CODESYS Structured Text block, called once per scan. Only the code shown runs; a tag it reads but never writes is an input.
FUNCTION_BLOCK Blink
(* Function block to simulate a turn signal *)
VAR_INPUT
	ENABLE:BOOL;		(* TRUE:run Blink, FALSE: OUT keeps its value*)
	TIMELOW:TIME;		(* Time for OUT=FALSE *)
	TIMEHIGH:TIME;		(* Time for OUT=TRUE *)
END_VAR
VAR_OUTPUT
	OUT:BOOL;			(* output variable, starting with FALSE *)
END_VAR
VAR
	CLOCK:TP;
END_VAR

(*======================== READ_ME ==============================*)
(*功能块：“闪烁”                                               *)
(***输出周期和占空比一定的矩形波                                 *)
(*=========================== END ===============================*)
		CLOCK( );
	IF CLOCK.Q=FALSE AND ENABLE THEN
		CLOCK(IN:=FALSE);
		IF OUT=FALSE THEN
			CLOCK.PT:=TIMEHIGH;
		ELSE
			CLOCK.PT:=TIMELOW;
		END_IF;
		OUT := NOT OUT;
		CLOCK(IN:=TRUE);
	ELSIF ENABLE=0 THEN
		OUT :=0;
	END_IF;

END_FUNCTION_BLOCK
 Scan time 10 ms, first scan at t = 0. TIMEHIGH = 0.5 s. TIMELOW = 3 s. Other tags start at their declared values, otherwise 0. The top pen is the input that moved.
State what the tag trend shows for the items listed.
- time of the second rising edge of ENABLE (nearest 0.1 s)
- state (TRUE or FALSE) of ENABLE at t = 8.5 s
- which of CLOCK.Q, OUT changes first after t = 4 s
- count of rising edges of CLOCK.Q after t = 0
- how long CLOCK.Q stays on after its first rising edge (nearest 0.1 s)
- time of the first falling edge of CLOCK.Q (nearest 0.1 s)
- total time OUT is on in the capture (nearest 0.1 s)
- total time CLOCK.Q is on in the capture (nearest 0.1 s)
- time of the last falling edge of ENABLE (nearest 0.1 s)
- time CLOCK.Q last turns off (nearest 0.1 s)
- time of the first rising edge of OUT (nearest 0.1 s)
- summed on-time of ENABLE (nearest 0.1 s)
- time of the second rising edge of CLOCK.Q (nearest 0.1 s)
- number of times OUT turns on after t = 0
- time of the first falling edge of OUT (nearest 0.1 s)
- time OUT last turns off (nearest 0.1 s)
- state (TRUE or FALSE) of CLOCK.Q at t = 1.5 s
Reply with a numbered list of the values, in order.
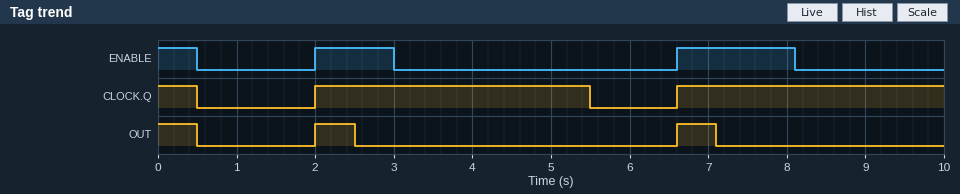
1. 6.6 s
2. FALSE
3. CLOCK.Q
4. 2
5. 3.5 s
6. 0.5 s
7. 1.5 s
8. 7.4 s
9. 8.1 s
10. 5.5 s
11. 2.0 s
12. 3.0 s
13. 6.6 s
14. 2
15. 0.5 s
16. 7.1 s
17. FALSE
